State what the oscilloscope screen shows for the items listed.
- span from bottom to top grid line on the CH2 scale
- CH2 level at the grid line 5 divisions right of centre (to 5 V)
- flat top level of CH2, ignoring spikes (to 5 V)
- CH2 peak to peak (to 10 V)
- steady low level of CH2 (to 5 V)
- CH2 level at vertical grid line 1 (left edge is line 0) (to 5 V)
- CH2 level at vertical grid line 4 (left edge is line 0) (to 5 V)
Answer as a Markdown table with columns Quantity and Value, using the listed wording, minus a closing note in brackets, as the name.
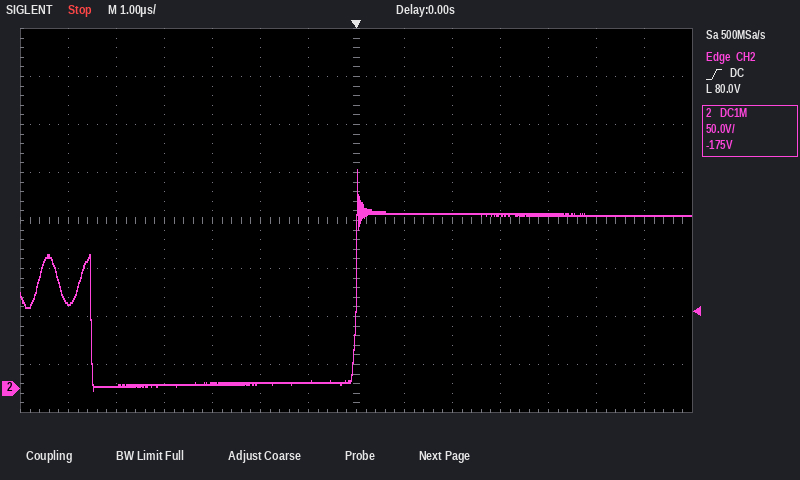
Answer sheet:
| Quantity | Value |
|---|---|
| span from bottom to top grid line on the CH2 scale | 400 V |
| CH2 level at the grid line 5 divisions right of centre | 180 V |
| flat top level of CH2, ignoring spikes | 180 V |
| CH2 peak to peak | 230 V |
| steady low level of CH2 | 5 V |
| CH2 level at vertical grid line 1 (left edge is line 0) | 90 V |
| CH2 level at vertical grid line 4 (left edge is line 0) | 5 V |
